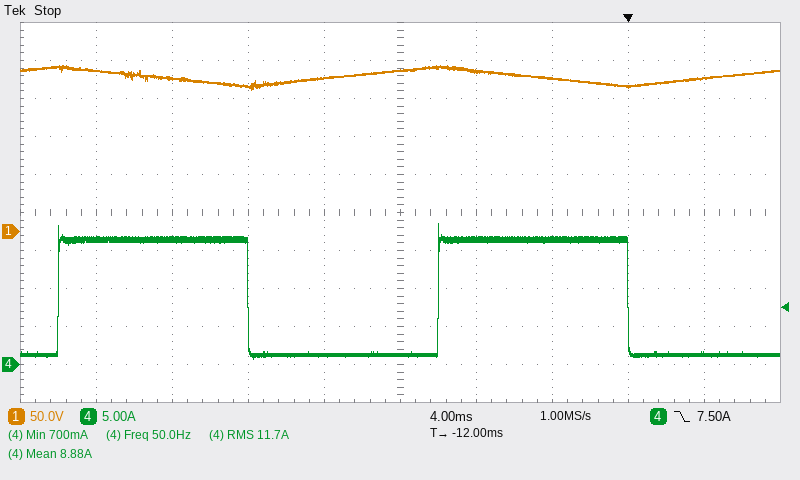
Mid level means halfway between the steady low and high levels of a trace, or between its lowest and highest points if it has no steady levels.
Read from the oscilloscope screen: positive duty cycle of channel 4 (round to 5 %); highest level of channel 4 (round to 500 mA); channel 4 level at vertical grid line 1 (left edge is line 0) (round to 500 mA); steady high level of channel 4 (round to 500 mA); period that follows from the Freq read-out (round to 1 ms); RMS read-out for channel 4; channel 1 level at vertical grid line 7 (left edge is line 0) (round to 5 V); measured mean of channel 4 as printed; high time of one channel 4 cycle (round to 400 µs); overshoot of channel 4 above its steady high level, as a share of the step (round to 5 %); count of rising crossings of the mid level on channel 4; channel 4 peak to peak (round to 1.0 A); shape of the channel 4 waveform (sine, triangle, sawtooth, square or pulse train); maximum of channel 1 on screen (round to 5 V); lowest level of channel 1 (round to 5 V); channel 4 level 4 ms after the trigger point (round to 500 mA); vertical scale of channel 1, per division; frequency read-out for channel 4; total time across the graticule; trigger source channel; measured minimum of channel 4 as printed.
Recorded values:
50 %
18.5 A
16.5 A
16.5 A
20 ms
11.7 A
200 V
8.88 A
10.0 ms
15 %
2
18.0 A
square
220 V
185 V
1.5 A
50 V
50.0 Hz
40 ms
channel 4
700 mA
